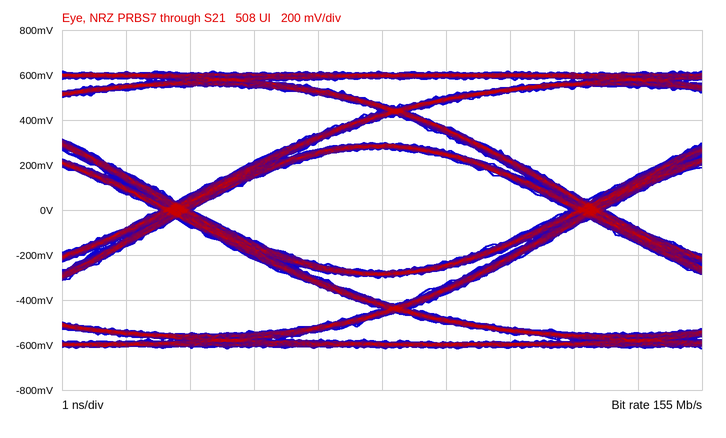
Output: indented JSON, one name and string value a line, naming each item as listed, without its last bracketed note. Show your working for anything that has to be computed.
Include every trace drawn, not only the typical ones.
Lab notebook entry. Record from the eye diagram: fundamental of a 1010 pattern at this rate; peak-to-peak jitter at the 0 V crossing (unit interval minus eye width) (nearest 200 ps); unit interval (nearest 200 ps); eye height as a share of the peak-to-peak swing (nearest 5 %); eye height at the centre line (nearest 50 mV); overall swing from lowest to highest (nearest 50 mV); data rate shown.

{
  "fundamental of a 1010 pattern at this rate": "77.5 MHz",
  "peak-to-peak jitter at the 0 V crossing (unit interval minus eye width)": "600 ps",
  "unit interval": "6.4 ns",
  "eye height as a share of the peak-to-peak swing": "550 mV / 1.25 V ≈ 44.0 %, so 45 % to the nearest 5 %",
  "eye height at the centre line": "550 mV",
  "overall swing from lowest to highest": "1.25 V",
  "data rate shown": "155 Mb/s"
}
